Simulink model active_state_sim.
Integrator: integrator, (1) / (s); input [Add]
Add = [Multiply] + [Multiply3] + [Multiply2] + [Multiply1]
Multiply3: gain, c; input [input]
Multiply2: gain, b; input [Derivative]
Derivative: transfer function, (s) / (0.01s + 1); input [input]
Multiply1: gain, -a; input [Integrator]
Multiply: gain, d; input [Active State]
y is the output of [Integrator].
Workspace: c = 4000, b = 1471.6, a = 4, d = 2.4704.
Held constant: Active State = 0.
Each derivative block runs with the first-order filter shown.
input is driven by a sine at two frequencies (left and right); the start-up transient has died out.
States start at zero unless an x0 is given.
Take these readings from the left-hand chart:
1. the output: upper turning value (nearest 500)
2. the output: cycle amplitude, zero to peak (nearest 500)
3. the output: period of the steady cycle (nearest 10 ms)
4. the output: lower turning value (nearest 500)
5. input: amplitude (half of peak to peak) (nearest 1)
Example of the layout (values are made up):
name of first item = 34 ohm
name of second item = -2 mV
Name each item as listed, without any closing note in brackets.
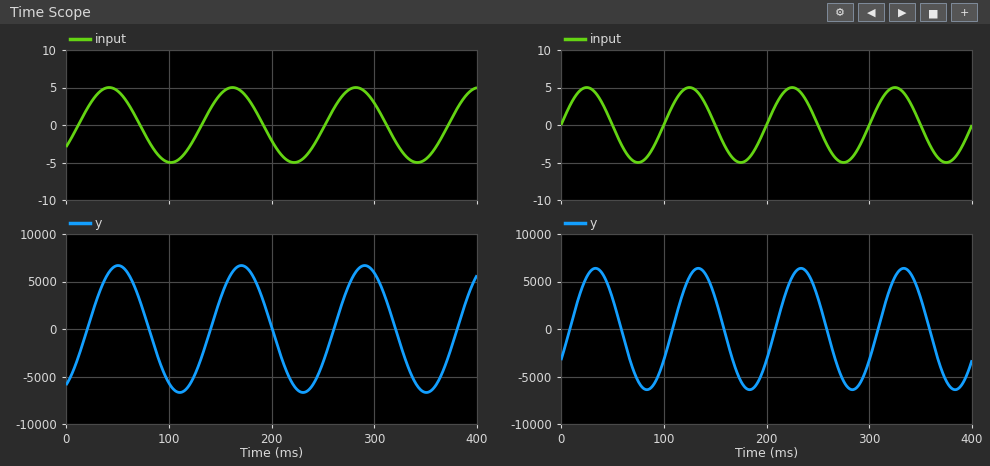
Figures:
the output: upper turning value = 6500
the output: cycle amplitude, zero to peak = 6500
the output: period of the steady cycle = 120 ms
the output: lower turning value = -6500
input: amplitude (half of peak to peak) = 5
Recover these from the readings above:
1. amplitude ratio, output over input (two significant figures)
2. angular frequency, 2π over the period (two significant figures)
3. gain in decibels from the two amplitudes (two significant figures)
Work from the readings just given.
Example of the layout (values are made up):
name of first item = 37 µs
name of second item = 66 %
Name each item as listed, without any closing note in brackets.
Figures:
amplitude ratio, output over input = 1300
angular frequency, 2π over the period = 0.052 rad/ms
gain in decibels from the two amplitudes = 62 dB
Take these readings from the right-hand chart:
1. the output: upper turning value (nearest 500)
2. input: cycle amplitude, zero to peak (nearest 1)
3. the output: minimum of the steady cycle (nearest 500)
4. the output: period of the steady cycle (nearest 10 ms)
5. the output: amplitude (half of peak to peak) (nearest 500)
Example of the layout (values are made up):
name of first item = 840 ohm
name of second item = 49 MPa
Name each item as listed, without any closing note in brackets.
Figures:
the output: upper turning value = 6500
input: cycle amplitude, zero to peak = 5
the output: minimum of the steady cycle = -6500
the output: period of the steady cycle = 100 ms
the output: amplitude (half of peak to peak) = 6500
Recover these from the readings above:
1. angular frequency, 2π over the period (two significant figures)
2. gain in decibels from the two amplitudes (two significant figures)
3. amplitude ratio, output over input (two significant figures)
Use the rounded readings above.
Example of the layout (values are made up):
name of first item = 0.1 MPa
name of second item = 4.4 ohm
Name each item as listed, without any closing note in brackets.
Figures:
angular frequency, 2π over the period = 0.063 rad/ms
gain in decibels from the two amplitudes = 62 dB
amplitude ratio, output over input = 1300
